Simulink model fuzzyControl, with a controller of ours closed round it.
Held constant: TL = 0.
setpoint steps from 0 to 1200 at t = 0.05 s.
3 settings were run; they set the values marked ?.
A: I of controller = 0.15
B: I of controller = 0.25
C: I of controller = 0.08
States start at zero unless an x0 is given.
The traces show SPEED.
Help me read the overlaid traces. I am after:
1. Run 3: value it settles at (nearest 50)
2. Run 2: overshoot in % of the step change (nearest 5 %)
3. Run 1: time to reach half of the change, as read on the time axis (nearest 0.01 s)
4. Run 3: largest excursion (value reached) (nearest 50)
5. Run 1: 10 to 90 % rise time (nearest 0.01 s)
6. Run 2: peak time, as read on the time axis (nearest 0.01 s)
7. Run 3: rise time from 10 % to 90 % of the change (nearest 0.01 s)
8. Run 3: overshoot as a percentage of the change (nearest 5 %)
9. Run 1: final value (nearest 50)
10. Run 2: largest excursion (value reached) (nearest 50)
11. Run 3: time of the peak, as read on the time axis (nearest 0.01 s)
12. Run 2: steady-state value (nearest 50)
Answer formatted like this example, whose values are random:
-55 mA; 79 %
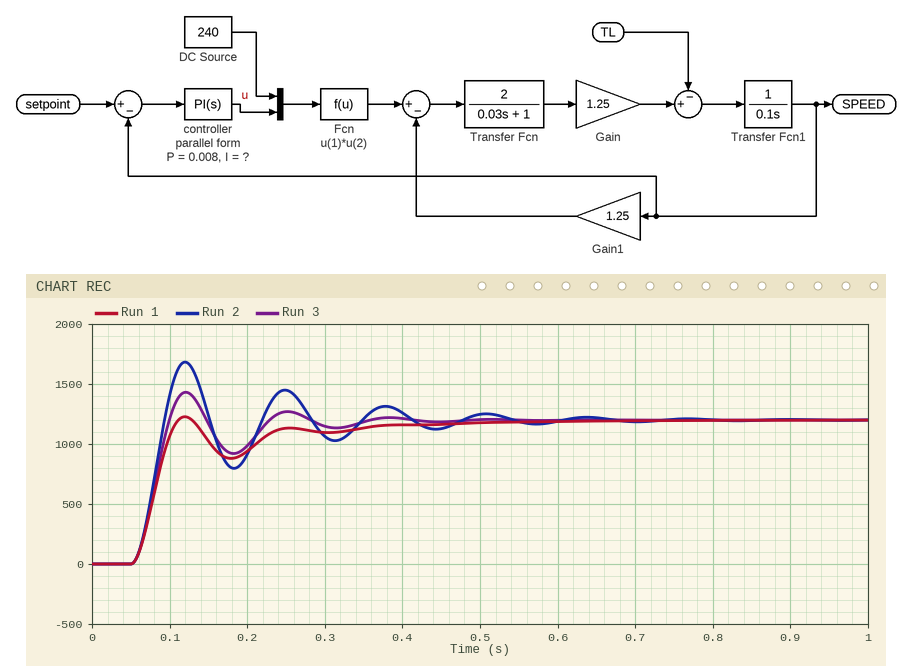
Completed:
1200; 40 %; 0.08 s; 1450; 0.04 s; 0.12 s; 0.03 s; 20 %; 1200; 1700; 0.12 s; 1200
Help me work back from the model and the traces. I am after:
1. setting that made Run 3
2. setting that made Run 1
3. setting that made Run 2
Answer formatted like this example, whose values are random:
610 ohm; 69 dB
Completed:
A; C; B
